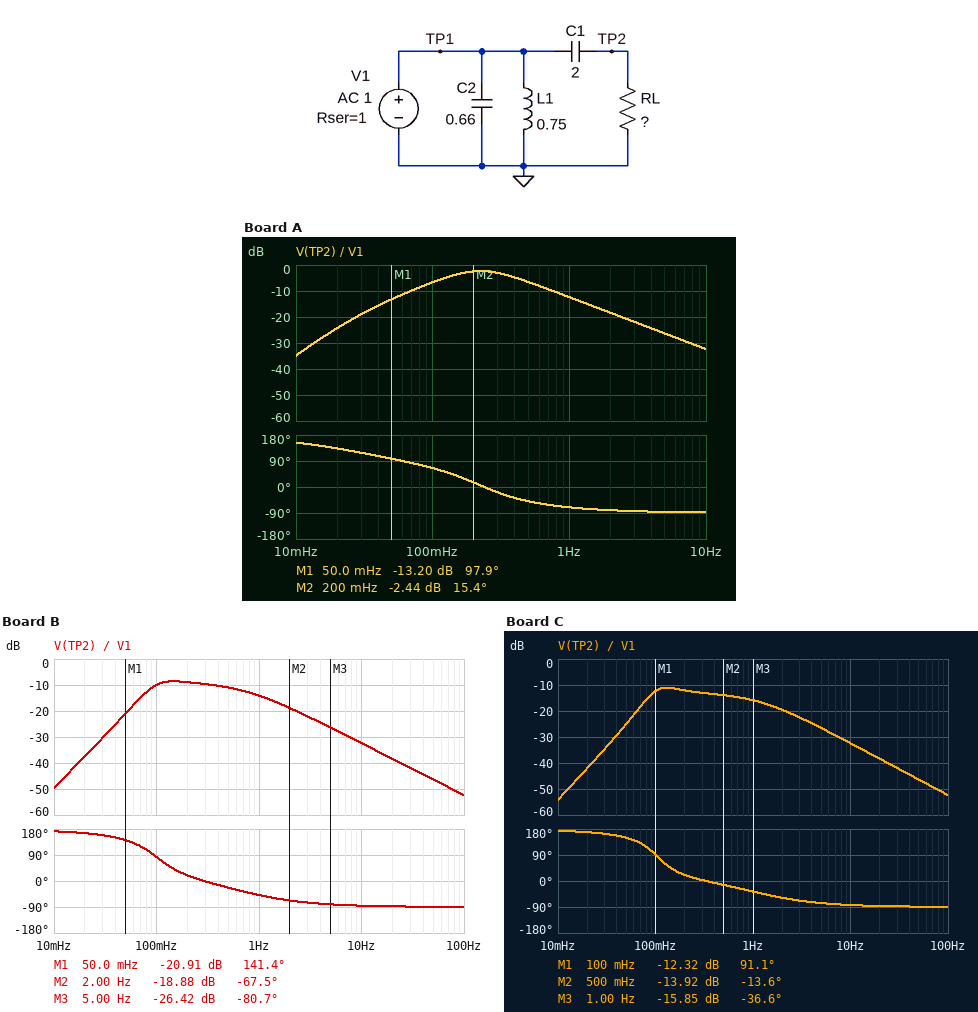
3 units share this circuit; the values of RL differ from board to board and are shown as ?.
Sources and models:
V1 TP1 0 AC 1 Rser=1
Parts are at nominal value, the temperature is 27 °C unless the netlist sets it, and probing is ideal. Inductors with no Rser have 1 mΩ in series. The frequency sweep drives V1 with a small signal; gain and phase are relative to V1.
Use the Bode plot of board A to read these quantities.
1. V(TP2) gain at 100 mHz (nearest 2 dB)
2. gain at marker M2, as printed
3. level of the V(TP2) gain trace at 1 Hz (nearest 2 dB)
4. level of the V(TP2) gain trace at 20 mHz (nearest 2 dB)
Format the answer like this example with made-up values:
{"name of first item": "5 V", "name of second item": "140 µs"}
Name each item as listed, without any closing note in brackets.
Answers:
{"V(TP2) gain at 100 mHz": "-6 dB", "gain at marker M2, as printed": "-2.44 dB", "level of the V(TP2) gain trace at 1 Hz": "-12 dB", "level of the V(TP2) gain trace at 20 mHz": "-24 dB"}
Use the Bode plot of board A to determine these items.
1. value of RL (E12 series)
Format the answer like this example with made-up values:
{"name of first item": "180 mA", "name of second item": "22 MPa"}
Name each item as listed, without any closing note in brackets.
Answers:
{"value of RL": "3.3 Ω"}
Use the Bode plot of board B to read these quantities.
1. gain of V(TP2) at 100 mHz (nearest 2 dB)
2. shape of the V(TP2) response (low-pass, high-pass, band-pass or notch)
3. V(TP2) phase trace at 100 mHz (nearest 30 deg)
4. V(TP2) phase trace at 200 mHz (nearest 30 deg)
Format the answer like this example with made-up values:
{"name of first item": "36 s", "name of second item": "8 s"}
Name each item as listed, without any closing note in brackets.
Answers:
{"gain of V(TP2) at 100 mHz": "-10 dB", "shape of the V(TP2) response": "band-pass", "V(TP2) phase trace at 100 mHz": "90 deg", "V(TP2) phase trace at 200 mHz": "30 deg"}
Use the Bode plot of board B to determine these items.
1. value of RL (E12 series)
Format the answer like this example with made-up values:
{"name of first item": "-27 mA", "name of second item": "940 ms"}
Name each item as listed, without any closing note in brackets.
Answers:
{"value of RL": "0.56 Ω"}
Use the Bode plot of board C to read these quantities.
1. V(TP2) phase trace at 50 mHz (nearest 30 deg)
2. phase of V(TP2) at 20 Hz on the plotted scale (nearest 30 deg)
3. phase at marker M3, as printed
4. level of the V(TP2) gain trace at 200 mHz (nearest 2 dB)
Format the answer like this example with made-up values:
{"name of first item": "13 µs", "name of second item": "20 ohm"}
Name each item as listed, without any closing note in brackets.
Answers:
{"V(TP2) phase trace at 50 mHz": "150 deg", "phase of V(TP2) at 20 Hz on the plotted scale": "-90 deg", "phase at marker M3, as printed": "-36.6 deg", "level of the V(TP2) gain trace at 200 mHz": "-12 dB"}
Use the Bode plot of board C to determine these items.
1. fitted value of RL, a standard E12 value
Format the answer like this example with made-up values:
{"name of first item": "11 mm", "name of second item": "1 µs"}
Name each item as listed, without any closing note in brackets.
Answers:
{"fitted value of RL, a standard E12 value": "0.33 Ω"}
